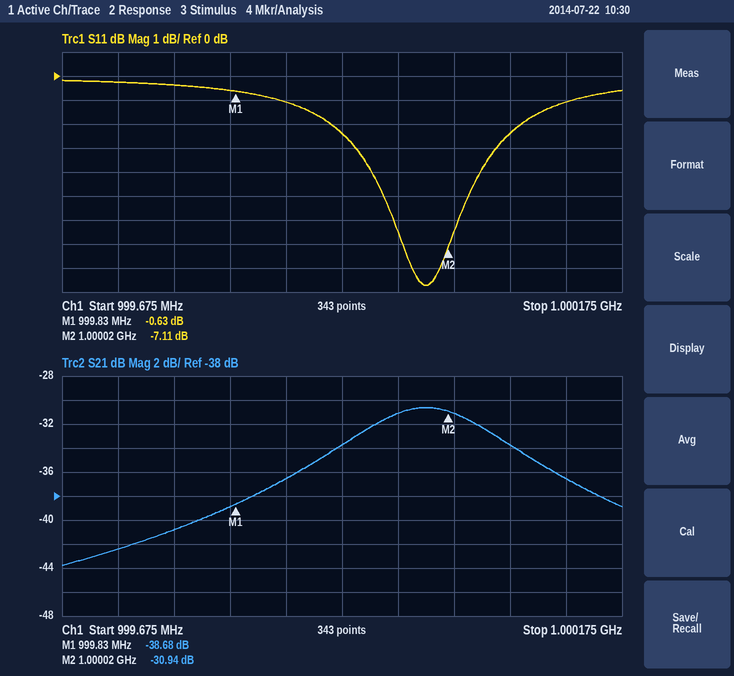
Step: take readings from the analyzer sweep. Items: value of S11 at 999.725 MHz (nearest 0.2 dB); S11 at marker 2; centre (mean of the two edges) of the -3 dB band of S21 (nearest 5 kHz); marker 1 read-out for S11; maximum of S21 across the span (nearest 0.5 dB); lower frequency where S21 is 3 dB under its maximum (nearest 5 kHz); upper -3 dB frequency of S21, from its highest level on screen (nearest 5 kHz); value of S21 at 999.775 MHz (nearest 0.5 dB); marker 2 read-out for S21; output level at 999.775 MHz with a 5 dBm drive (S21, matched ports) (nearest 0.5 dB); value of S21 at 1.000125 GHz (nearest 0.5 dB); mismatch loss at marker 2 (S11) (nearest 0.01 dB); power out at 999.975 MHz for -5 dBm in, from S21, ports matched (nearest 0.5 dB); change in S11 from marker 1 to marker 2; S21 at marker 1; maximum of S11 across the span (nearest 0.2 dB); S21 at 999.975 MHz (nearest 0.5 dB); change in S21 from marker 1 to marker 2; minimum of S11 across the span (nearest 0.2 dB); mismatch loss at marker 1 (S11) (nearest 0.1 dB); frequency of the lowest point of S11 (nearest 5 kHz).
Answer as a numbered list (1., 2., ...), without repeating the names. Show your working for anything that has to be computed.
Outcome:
1. -0.2 dB
2. -7.11 dB
3. 1.000000 GHz
4. -0.63 dB
5. -30.5 dB
6. 999.925 MHz
7. 1.000075 GHz
8. -41.0 dB
9. -30.94 dB
10. 5 dBm + (-41.0 dB) = -36.0 dBm
11. -36.5 dB
12. −10 log10(1 − 10^(-7.11/10)) ≈ 0.94 dB
13. -5 dBm + (-31.0 dB) = -36.0 dBm
14. -7.11 − (-0.63) = -6.48 dB
15. -38.68 dB
16. -0.2 dB
17. -31.0 dB
18. -30.94 − (-38.68) = 7.74 dB
19. -8.8 dB
20. −10 log10(1 − 10^(-0.63/10)) ≈ 8.7 dB
21. 1.000000 GHz
